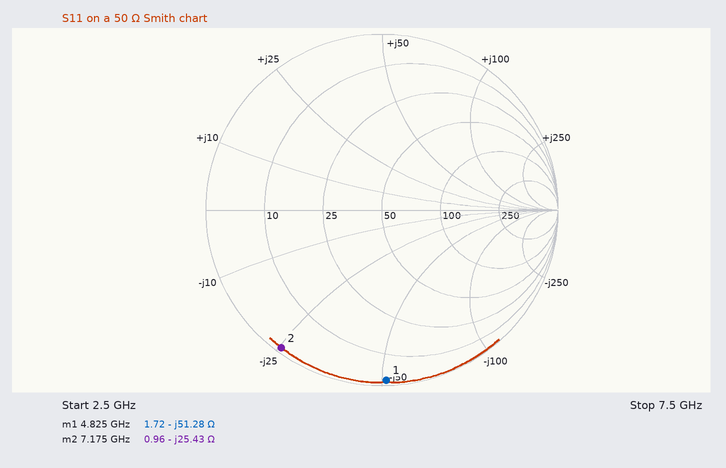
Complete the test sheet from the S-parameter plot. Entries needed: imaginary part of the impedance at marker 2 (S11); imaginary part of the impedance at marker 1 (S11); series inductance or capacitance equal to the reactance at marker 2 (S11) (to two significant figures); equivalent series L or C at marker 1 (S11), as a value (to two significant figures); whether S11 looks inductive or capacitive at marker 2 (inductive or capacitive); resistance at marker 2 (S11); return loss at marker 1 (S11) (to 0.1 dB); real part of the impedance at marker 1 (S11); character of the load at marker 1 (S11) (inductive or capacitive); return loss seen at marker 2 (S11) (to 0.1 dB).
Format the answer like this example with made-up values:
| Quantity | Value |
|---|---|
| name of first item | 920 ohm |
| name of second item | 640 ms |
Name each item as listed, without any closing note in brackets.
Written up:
| Quantity | Value |
|---|---|
| imaginary part of the impedance at marker 2 | -25.43 Ω |
| imaginary part of the impedance at marker 1 | -51.28 Ω |
| series inductance or capacitance equal to the reactance at marker 2 (S11) | 870 fF |
| equivalent series L or C at marker 1 (S11), as a value | 640 fF |
| whether S11 looks inductive or capacitive at marker 2 | capacitive |
| resistance at marker 2 | 0.96 Ω |
| return loss at marker 1 (S11) | 0.3 dB |
| real part of the impedance at marker 1 | 1.72 Ω |
| character of the load at marker 1 (S11) | capacitive |
| return loss seen at marker 2 (S11) | 0.3 dB |
